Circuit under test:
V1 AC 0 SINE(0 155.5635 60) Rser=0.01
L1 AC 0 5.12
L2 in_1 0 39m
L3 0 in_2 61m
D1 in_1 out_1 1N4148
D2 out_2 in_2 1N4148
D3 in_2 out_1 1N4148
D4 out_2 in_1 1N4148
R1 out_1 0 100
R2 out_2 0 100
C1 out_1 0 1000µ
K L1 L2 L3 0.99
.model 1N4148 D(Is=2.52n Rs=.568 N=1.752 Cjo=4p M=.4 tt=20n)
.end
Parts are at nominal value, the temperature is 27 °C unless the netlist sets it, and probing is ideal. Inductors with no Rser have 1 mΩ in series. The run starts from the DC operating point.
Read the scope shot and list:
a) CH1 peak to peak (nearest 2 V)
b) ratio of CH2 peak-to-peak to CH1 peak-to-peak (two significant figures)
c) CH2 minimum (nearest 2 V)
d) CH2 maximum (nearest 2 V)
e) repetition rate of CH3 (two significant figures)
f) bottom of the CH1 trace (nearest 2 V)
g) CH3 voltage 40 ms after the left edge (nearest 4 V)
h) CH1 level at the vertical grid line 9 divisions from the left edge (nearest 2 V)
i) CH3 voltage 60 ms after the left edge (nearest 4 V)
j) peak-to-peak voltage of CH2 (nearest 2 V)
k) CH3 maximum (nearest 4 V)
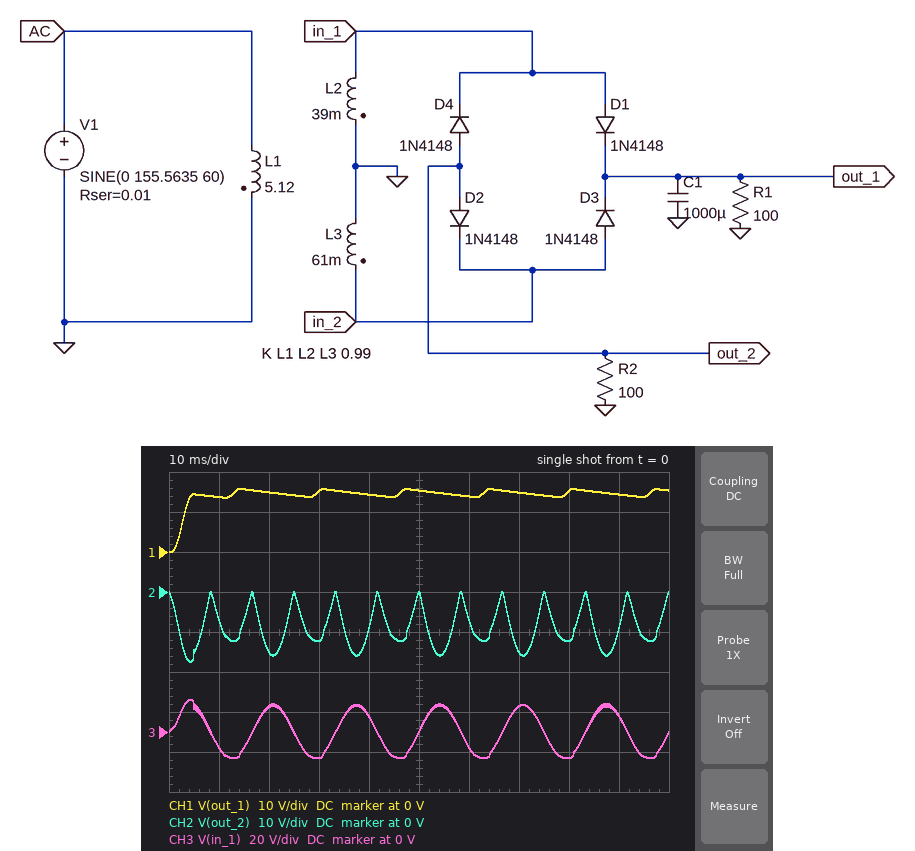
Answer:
16 V
1.1
-18 V
0 V
60 Hz
0 V
8 V
14 V
-8 V
18 V
16 V
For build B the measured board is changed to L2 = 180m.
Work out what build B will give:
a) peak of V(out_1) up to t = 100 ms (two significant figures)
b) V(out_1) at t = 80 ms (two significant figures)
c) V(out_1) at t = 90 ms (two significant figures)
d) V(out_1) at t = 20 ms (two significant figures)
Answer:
39 V
25 V
26 V
34 V
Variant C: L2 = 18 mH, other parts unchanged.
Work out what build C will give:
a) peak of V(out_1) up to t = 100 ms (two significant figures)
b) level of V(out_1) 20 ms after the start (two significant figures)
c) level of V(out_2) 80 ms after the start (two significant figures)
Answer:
18 V
17 V
-8.1 V
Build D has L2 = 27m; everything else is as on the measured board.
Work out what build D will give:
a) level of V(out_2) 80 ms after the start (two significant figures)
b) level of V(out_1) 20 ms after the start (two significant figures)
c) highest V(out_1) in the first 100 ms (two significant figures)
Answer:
-10 V
16 V
17 V
